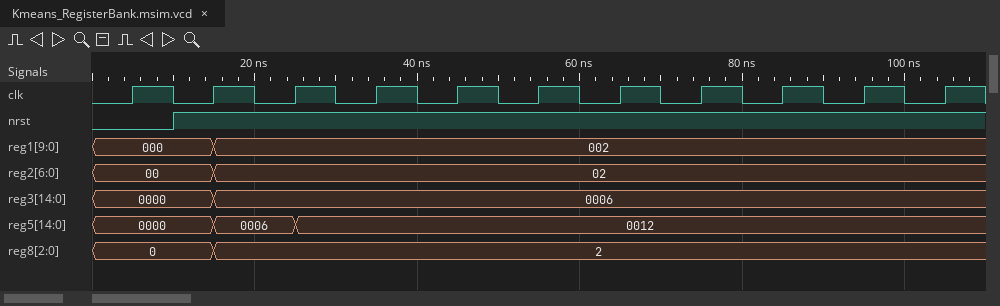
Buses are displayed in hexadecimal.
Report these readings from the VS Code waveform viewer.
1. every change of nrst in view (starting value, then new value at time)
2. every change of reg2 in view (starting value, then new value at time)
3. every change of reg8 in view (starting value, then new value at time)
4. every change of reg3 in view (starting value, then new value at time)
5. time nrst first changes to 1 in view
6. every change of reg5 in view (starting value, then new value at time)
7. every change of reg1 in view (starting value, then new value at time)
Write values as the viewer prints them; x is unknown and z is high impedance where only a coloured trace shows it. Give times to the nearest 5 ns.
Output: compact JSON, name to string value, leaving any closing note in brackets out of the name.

{"every change of nrst in view": "0, 1 at 10 ns", "every change of reg2 in view": "00, 02 at 15 ns", "every change of reg8 in view": "0, 2 at 15 ns", "every change of reg3 in view": "0000, 0006 at 15 ns", "time nrst first changes to 1 in view": "10 ns", "every change of reg5 in view": "0000, 0006 at 15 ns, 0012 at 25 ns", "every change of reg1 in view": "000, 002 at 15 ns"}
